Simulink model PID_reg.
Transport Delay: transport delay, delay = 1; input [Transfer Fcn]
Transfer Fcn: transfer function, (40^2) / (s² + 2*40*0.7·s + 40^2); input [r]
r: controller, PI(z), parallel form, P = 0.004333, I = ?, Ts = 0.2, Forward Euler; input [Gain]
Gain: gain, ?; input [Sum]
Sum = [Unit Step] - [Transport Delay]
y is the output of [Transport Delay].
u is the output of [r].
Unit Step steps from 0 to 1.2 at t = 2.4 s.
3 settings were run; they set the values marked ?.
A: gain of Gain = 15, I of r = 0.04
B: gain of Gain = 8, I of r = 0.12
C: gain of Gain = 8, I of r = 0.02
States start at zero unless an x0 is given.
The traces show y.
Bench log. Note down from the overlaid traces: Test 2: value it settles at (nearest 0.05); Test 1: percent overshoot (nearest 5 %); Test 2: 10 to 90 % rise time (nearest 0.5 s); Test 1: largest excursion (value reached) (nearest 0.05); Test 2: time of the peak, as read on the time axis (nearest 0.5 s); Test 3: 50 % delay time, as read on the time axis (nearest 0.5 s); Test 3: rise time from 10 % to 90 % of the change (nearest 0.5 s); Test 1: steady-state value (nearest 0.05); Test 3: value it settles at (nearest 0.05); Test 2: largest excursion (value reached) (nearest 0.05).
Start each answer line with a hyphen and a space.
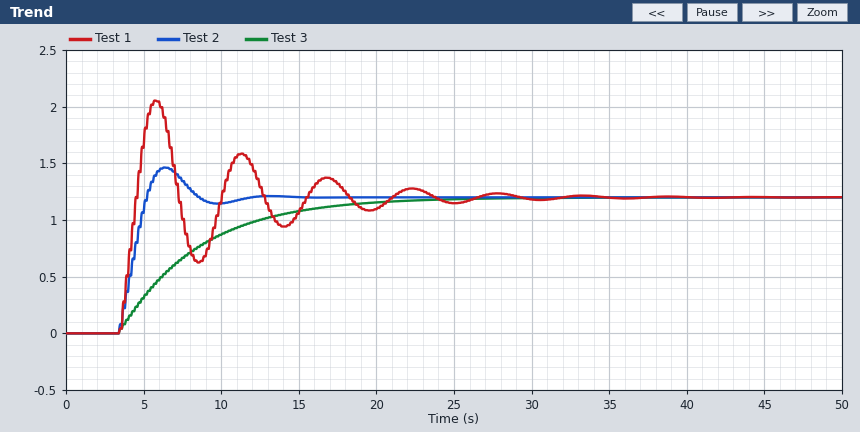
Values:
- 1.20
- 70 %
- 1.5 s
- 2.05
- 6.5 s
- 7.0 s
- 11.0 s
- 1.20
- 1.20
- 1.45
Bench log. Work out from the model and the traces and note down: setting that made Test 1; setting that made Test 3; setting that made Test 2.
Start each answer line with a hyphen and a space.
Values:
- B
- C
- A
